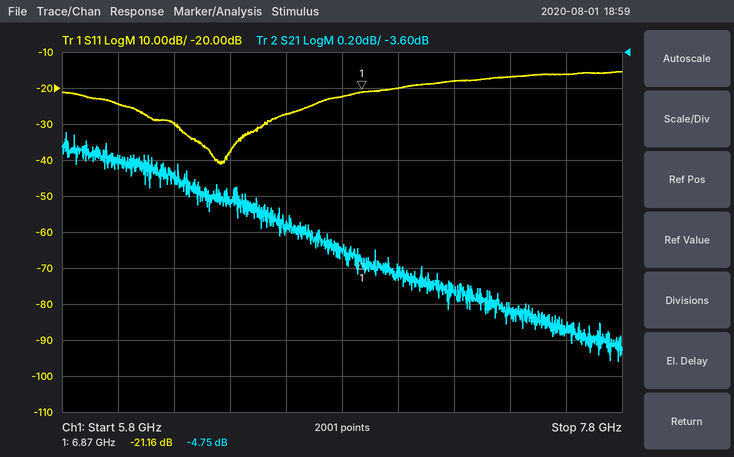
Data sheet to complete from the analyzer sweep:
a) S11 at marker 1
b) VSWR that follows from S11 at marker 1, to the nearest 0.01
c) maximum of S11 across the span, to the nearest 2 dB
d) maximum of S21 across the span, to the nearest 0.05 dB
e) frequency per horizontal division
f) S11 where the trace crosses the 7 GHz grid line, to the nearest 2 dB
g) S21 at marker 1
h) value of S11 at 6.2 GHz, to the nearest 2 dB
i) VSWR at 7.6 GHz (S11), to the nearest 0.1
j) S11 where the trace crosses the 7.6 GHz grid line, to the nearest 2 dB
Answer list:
-21.16 dB
1.19
-16 dB
-4.05 dB
200 MHz
-20 dB
-4.75 dB
-30 dB
1.4
-16 dB
